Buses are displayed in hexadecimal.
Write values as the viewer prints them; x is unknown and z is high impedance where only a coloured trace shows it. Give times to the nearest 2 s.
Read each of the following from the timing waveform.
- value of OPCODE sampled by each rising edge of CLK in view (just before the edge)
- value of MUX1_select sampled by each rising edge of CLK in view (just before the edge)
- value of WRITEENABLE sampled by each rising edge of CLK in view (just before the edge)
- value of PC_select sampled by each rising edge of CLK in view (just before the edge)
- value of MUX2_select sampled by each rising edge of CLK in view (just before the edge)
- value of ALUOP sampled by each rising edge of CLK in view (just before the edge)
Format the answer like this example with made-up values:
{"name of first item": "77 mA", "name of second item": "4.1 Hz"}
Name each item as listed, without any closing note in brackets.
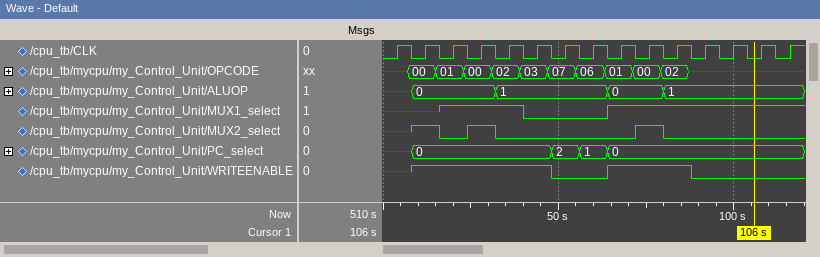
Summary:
{"value of OPCODE sampled by each rising edge of CLK in view": "x, 00, 01, 00, 02, 03, 07, 06, 01, 00, 02, x, x, x, x", "value of MUX1_select sampled by each rising edge of CLK in view": "x x 1 1 1 0 0 0 1 1 1 1 1 1 1", "value of WRITEENABLE sampled by each rising edge of CLK in view": "x 1 1 1 1 1 0 0 1 1 1 0 0 0 0", "value of PC_select sampled by each rising edge of CLK in view": "x, 0, 0, 0, 0, 0, 2, 1, 0, 0, 0, 0, 0, 0, 0", "value of MUX2_select sampled by each rising edge of CLK in view": "x 1 0 1 0 0 0 0 0 1 0 0 0 0 0", "value of ALUOP sampled by each rising edge of CLK in view": "x, 0, 0, 0, 1, 1, 1, 1, 0, 0, 1, 1, 1, 1, 1"}
